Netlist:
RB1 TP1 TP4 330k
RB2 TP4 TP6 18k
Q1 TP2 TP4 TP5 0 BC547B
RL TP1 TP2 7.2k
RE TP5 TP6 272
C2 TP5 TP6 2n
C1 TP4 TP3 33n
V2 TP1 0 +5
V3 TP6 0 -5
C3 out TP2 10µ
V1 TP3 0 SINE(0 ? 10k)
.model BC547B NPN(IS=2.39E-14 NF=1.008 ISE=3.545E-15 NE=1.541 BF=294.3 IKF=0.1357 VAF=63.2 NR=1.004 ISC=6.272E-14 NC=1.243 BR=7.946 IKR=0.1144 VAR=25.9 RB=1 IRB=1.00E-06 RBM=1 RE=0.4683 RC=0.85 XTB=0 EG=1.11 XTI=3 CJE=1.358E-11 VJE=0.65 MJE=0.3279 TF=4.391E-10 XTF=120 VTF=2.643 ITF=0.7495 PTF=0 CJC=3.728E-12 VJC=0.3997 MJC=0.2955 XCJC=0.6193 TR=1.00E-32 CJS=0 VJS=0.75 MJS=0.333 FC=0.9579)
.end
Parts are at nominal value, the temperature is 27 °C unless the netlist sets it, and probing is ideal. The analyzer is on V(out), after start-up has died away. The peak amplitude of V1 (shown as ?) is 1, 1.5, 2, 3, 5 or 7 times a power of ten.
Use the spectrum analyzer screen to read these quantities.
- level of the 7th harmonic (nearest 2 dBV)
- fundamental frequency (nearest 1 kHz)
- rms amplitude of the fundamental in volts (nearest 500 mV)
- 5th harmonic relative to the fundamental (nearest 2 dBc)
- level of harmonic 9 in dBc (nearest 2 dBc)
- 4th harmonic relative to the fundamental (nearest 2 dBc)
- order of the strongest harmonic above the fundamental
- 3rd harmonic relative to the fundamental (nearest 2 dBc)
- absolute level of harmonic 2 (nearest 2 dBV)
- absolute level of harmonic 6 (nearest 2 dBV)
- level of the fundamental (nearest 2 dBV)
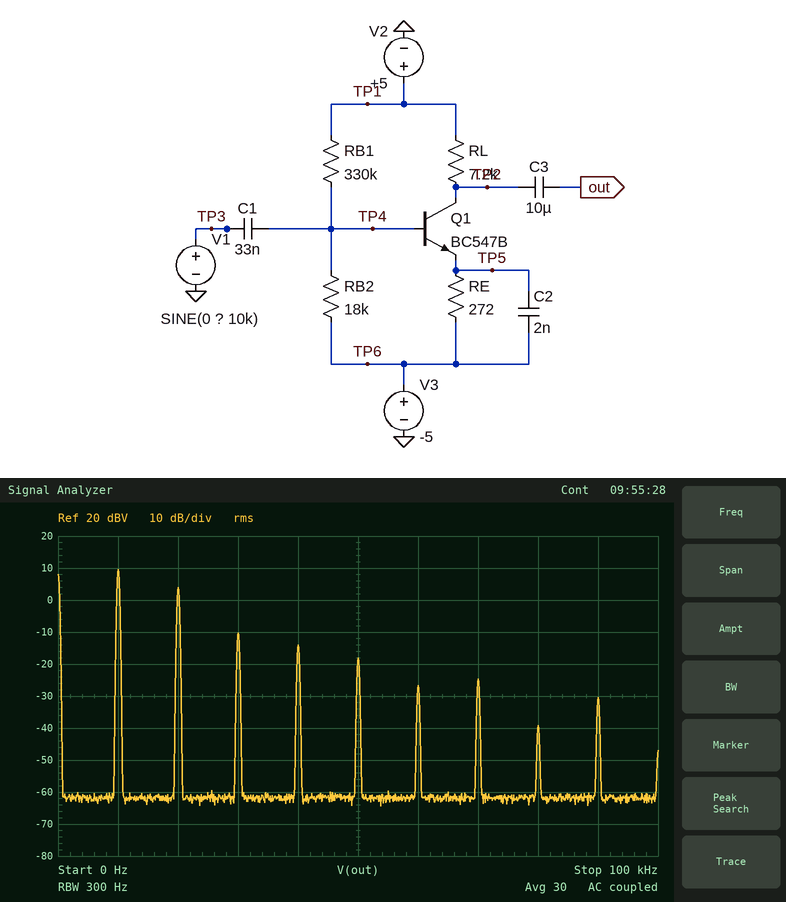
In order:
-24 dBV
10 kHz
3.0 V
-28 dBc
-40 dBc
-24 dBc
2
-20 dBc
4 dBV
-26 dBV
10 dBV
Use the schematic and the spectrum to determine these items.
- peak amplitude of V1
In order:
500 mV
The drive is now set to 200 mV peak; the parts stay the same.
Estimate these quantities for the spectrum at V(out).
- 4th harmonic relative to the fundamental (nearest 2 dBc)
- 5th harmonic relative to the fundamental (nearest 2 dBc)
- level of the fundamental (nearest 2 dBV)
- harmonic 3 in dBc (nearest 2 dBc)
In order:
-30 dBc
-30 dBc
-2 dBV
-18 dBc
